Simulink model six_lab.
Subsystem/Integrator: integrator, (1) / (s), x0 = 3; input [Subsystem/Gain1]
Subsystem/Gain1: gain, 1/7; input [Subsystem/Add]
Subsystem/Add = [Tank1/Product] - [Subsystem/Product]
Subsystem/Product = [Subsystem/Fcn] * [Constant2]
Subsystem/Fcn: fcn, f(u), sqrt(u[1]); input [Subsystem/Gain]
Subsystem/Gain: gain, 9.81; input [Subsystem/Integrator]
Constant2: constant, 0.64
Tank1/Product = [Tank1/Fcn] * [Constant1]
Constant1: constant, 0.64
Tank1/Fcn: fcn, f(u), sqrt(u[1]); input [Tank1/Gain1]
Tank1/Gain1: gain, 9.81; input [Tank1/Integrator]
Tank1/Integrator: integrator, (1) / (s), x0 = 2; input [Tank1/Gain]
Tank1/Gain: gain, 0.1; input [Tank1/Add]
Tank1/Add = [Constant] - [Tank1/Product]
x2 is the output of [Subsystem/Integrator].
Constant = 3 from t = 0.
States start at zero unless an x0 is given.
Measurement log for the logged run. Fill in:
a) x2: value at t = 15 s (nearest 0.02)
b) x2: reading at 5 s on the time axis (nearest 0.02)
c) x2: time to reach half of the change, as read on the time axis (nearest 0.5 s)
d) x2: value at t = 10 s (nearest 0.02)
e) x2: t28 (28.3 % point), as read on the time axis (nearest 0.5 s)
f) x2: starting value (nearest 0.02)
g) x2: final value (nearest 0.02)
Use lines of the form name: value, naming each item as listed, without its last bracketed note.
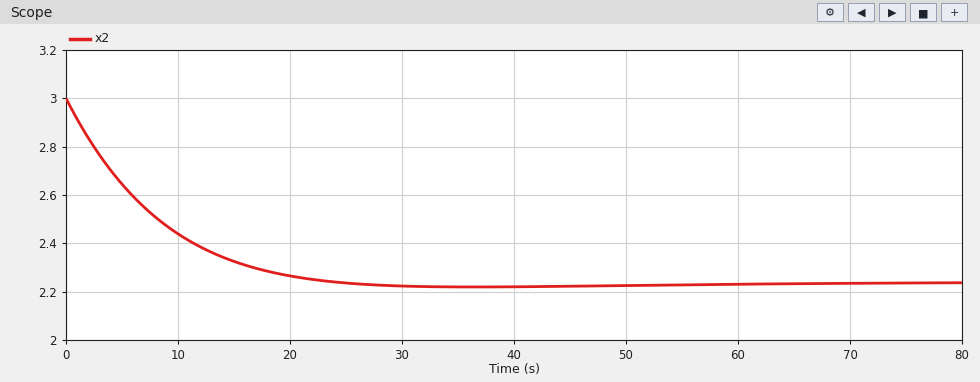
x2: value at t = 15 s: 2.32
x2: reading at 5 s on the time axis: 2.64
x2: time to reach half of the change, as read on the time axis: 5.5 s
x2: value at t = 10 s: 2.44
x2: t28 (28.3 % point), as read on the time axis: 2.5 s
x2: starting value: 3.00
x2: final value: 2.24
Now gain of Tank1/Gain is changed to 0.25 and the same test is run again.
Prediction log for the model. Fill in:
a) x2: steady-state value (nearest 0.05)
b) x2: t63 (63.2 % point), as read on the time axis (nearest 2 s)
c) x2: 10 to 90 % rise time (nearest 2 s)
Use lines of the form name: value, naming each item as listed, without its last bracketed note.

x2: steady-state value: 2.25
x2: t63 (63.2 % point), as read on the time axis: 8 s
x2: 10 to 90 % rise time: 20 s
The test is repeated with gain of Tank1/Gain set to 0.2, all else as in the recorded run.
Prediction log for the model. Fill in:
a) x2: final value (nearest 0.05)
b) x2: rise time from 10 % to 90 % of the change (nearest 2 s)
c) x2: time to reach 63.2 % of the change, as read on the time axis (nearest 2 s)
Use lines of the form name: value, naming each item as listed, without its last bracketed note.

x2: final value: 2.25
x2: rise time from 10 % to 90 % of the change: 18 s
x2: time to reach 63.2 % of the change, as read on the time axis: 8 s
